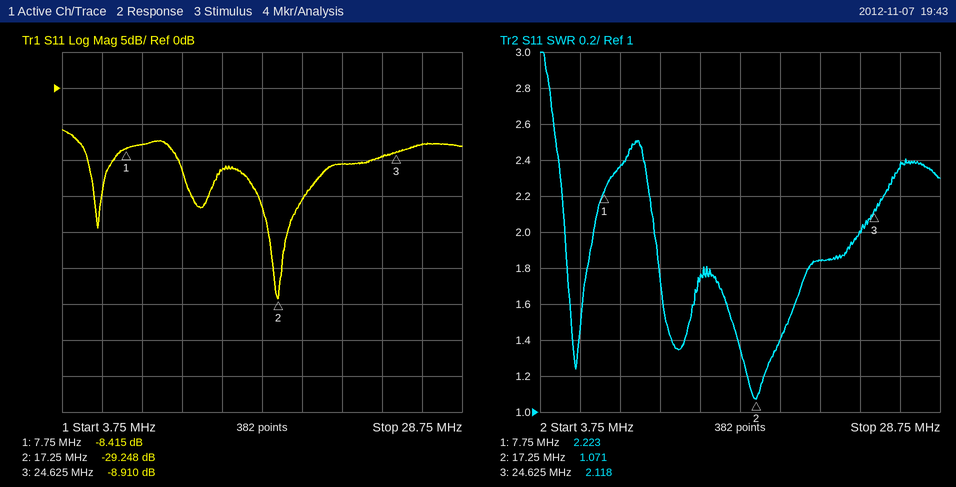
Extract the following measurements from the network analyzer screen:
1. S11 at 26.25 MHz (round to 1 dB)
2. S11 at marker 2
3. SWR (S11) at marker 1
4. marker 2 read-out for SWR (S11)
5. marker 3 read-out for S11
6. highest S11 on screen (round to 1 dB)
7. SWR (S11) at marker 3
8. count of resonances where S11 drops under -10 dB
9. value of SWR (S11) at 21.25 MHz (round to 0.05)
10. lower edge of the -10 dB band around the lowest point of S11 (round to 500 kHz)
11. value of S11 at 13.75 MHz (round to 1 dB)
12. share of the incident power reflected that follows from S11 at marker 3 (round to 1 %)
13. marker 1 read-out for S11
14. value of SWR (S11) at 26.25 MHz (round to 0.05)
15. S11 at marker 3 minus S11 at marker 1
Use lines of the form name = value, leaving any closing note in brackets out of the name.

S11 at 26.25 MHz = -8 dB
S11 at marker 2 = -29.248 dB
SWR (S11) at marker 1 = 2.223
marker 2 read-out for SWR = 1.071
marker 3 read-out for S11 = -8.910 dB
highest S11 on screen = -6 dB
SWR (S11) at marker 3 = 2.118
count of resonances where S11 drops under -10 dB = 3
value of SWR (S11) at 21.25 MHz = 1.85
lower edge of the -10 dB band around the lowest point of S11 = 11.0 MHz
value of S11 at 13.75 MHz = -11 dB
share of the incident power reflected that follows from S11 at marker 3 = 13 %
marker 1 read-out for S11 = -8.415 dB
value of SWR (S11) at 26.25 MHz = 2.35
S11 at marker 3 minus S11 at marker 1 = -0.495 dB
